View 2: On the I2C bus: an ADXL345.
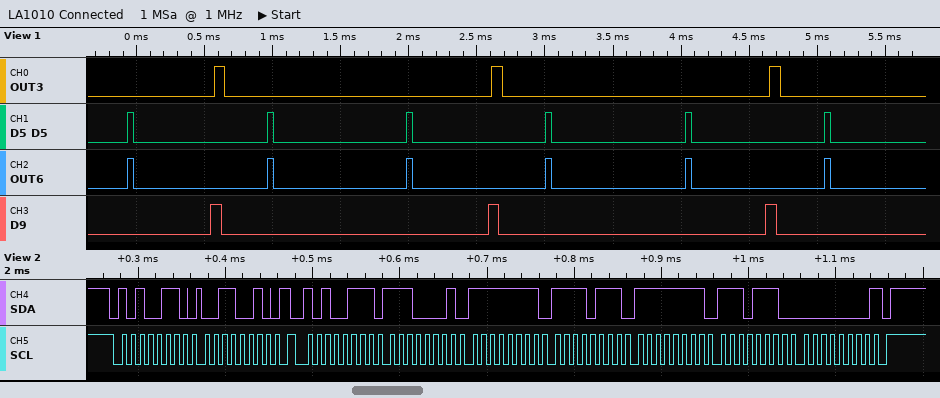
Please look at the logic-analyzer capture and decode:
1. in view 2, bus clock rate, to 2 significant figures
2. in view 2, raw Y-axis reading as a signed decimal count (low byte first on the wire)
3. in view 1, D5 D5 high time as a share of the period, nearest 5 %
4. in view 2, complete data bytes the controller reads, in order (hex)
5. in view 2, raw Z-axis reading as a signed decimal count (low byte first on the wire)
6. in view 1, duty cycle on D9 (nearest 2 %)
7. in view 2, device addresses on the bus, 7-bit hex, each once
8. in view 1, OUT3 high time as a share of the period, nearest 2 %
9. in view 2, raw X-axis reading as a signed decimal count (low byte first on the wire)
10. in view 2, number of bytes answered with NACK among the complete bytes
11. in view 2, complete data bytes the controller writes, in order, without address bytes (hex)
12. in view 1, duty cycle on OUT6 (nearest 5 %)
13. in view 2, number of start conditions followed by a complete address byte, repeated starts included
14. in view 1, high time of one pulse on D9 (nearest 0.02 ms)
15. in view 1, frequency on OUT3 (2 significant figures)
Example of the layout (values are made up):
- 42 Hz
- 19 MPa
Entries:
- 100 kHz
- -9
- 5 %
- E1 FF F7 FF EE 00
- 238
- 4 %
- 0x53
- 4 %
- -31
- 1
- 32
- 5 %
- 2
- 0.08 ms
- 490 Hz
